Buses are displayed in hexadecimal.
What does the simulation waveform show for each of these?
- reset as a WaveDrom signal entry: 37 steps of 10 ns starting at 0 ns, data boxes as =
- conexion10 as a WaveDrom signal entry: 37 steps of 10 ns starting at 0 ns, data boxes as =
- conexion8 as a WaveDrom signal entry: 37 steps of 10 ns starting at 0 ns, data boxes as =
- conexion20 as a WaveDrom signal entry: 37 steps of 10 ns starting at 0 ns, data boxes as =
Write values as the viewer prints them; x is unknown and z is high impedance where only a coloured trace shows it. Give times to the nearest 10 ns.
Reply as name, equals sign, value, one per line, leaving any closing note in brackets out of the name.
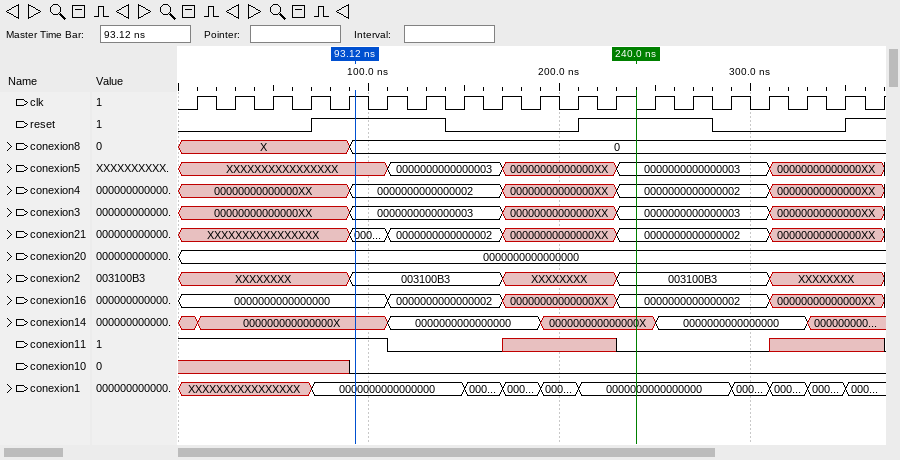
reset as a WaveDrom signal entry: 37 steps of 10 ns starting at 0 ns, data boxes as = = {name: 'reset', wave: '0......1......0......1......0......1.'}
conexion10 as a WaveDrom signal entry: 37 steps of 10 ns starting at 0 ns, data boxes as = = {name: 'conexion10', wave: 'x........0...........................'}
conexion8 as a WaveDrom signal entry: 37 steps of 10 ns starting at 0 ns, data boxes as = = {name: 'conexion8', wave: 'x........=...........................', data: '0'}
conexion20 as a WaveDrom signal entry: 37 steps of 10 ns starting at 0 ns, data boxes as = = {name: 'conexion20', wave: '=....................................', data: '0000000000000000'}
